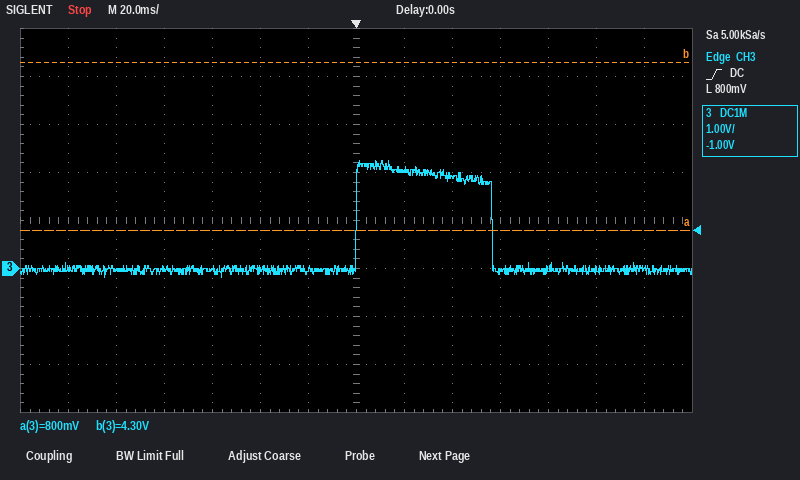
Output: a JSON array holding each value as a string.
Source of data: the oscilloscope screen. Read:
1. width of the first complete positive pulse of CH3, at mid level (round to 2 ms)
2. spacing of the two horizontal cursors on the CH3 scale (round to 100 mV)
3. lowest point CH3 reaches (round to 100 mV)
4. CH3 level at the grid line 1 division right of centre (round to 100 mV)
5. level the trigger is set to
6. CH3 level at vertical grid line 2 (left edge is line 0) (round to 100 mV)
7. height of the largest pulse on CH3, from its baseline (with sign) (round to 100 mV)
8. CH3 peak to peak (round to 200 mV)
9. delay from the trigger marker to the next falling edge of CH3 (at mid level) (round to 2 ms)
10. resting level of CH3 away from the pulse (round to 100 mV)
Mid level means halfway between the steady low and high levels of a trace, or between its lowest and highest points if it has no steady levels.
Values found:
["56 ms", "3.5 V", "-200 mV", "2.1 V", "800 mV", "0.0 V", "+2.3 V", "2.4 V", "56 ms", "0.0 V"]
